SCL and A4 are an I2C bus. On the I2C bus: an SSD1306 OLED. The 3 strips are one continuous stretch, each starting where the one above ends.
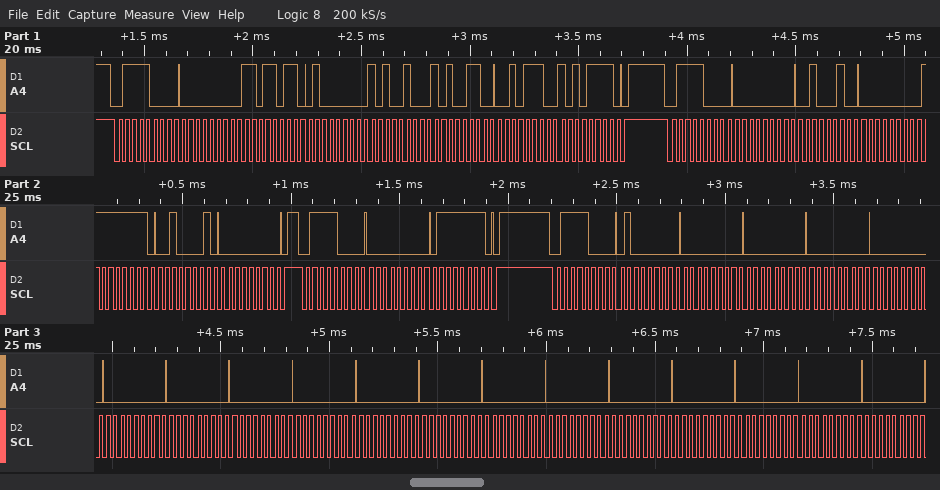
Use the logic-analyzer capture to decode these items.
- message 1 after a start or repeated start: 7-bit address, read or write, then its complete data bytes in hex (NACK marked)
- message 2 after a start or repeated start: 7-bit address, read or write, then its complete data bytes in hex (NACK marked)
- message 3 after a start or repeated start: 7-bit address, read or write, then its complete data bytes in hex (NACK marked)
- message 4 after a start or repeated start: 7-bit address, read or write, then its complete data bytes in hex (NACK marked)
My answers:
0x3C write: 00 DB 40 A4 A6 2E AF
0x3C write: 00 22 00 FF 21 00
0x3C write: 00 7F
0x3C write: 40 00 00 00 00 00 00 00 00 00 00 00 00 00 00 00 00 00
